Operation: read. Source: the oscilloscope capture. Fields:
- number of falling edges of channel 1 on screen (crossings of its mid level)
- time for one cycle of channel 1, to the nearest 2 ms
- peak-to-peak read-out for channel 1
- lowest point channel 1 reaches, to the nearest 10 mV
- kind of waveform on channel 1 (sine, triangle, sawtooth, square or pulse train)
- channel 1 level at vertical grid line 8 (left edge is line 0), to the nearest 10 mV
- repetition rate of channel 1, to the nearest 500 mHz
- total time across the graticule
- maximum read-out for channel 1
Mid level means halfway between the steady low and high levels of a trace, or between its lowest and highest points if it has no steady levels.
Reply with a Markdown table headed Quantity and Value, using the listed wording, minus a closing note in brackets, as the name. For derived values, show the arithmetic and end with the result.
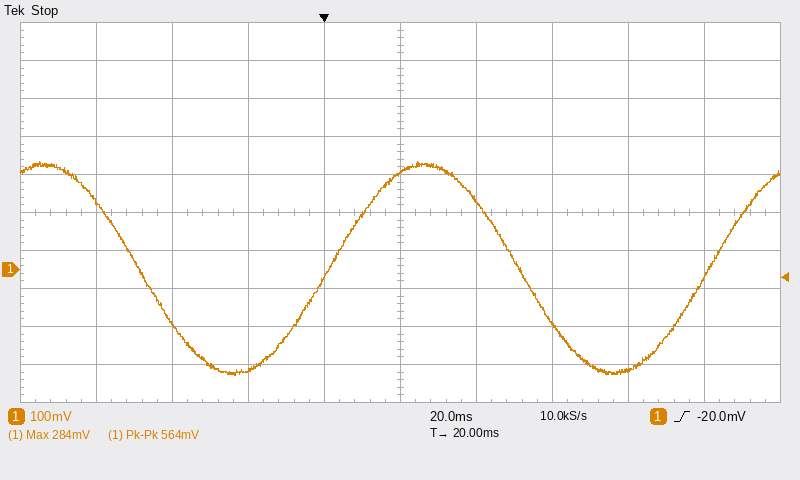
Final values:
| Quantity | Value |
|---|---|
| number of falling edges of channel 1 on screen | 2 |
| time for one cycle of channel 1, to the nearest 2 ms | 100 ms |
| peak-to-peak read-out for channel 1 | 564 mV |
| lowest point channel 1 reaches, to the nearest 10 mV | -280 mV |
| kind of waveform on channel 1 | sine |
| channel 1 level at vertical grid line 8 (left edge is line 0), to the nearest 10 mV | -270 mV |
| repetition rate of channel 1, to the nearest 500 mHz | 1 / 100 ms ≈ 10.0 Hz |
| total time across the graticule | 200 ms |
| maximum read-out for channel 1 | 284 mV |
